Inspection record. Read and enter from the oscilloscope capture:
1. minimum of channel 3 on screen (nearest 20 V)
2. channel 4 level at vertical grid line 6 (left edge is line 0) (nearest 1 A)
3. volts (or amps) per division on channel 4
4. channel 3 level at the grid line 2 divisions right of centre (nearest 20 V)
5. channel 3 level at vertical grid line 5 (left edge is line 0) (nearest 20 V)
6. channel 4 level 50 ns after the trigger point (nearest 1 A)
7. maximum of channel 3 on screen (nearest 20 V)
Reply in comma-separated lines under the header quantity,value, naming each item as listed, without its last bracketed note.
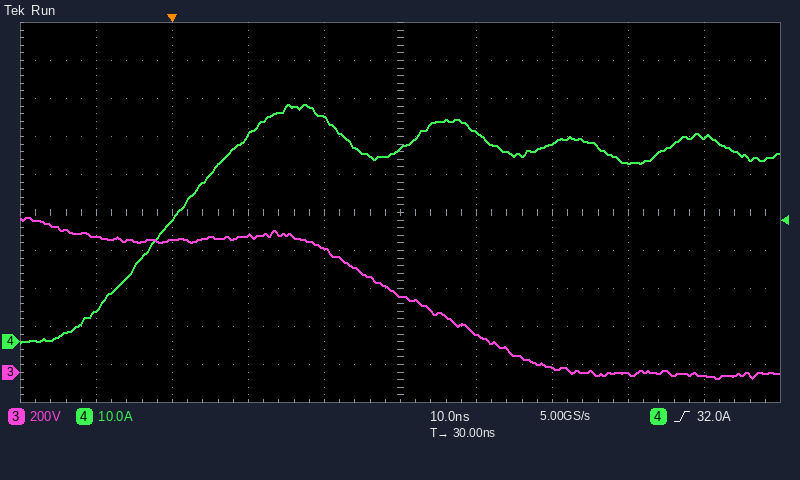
quantity,value
minimum of channel 3 on screen,-40 V
channel 4 level at vertical grid line 6 (left edge is line 0),55 A
volts (or amps) per division on channel 4,10 A
channel 3 level at the grid line 2 divisions right of centre,20 V
channel 3 level at vertical grid line 5 (left edge is line 0),400 V
channel 4 level 50 ns after the trigger point,52 A
maximum of channel 3 on screen,820 V
